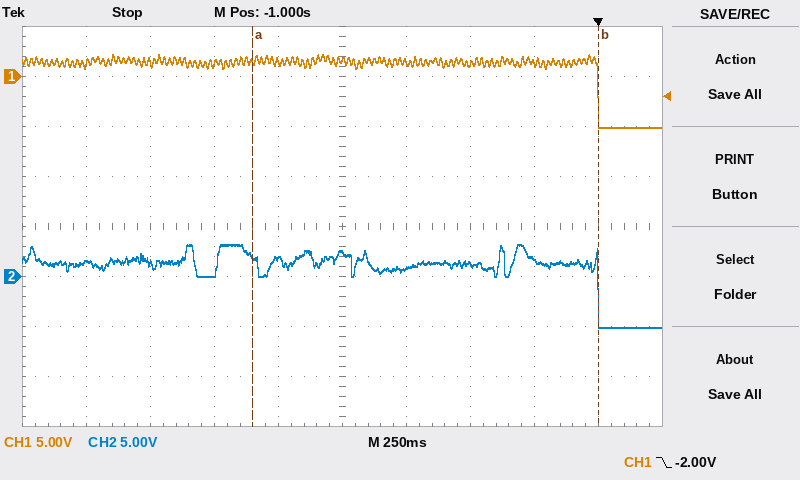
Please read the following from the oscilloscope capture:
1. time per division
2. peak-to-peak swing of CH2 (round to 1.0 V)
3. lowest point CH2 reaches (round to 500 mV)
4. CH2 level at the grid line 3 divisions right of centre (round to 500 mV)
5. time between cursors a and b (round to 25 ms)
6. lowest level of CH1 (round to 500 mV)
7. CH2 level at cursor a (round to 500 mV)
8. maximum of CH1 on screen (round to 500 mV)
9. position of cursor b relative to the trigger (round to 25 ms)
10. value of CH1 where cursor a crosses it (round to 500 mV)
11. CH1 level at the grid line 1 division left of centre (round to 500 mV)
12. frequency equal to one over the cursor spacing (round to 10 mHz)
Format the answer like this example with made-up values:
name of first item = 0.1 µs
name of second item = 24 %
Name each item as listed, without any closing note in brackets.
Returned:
time per division = 250 ms
peak-to-peak swing of CH2 = 8.0 V
lowest point CH2 reaches = -5.0 V
CH2 level at the grid line 3 divisions right of centre = 1.5 V
time between cursors a and b = 1.350 s
lowest level of CH1 = -5.0 V
CH2 level at cursor a = 2.0 V
maximum of CH1 on screen = 2.0 V
position of cursor b relative to the trigger = 0 ms
value of CH1 where cursor a crosses it = 1.5 V
CH1 level at the grid line 1 division left of centre = 1.5 V
frequency equal to one over the cursor spacing = 740 mHz
